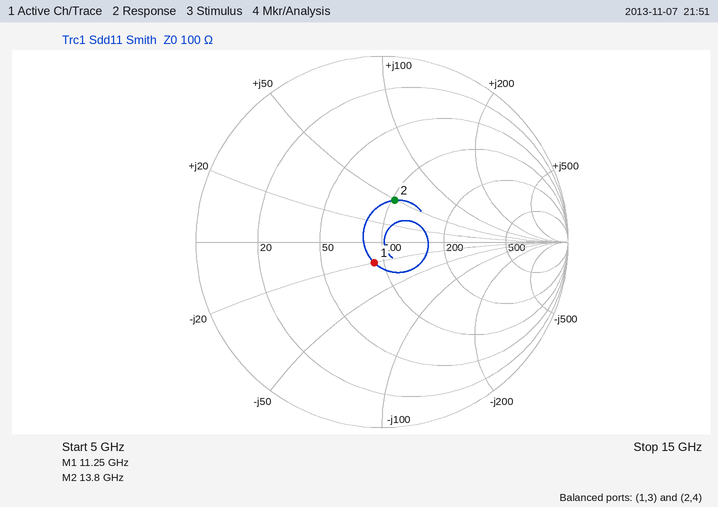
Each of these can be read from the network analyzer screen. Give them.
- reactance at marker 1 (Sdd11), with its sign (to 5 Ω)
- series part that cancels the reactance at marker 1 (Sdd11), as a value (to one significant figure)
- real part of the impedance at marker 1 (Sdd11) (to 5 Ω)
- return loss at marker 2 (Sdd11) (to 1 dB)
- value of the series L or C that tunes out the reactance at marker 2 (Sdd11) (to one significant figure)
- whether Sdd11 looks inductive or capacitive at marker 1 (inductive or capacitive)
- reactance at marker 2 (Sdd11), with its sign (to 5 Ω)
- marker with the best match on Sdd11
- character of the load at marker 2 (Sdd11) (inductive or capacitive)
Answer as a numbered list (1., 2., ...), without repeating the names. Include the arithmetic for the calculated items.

1. -20 Ω
2. L = 20 Ω/(2π × 11.25 GHz) ≈ 283 pH, so 300 pH to one significant figure
3. 90 Ω
4. 13 dB
5. C = 1/(2π × 13.8 GHz × 50 Ω) ≈ 231 fF, so 200 fF to one significant figure
6. capacitive
7. +50 Ω
8. marker 1
9. inductive
